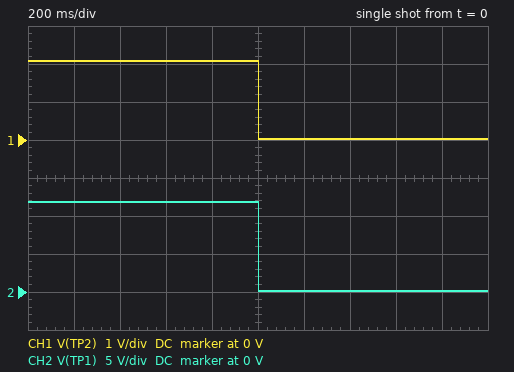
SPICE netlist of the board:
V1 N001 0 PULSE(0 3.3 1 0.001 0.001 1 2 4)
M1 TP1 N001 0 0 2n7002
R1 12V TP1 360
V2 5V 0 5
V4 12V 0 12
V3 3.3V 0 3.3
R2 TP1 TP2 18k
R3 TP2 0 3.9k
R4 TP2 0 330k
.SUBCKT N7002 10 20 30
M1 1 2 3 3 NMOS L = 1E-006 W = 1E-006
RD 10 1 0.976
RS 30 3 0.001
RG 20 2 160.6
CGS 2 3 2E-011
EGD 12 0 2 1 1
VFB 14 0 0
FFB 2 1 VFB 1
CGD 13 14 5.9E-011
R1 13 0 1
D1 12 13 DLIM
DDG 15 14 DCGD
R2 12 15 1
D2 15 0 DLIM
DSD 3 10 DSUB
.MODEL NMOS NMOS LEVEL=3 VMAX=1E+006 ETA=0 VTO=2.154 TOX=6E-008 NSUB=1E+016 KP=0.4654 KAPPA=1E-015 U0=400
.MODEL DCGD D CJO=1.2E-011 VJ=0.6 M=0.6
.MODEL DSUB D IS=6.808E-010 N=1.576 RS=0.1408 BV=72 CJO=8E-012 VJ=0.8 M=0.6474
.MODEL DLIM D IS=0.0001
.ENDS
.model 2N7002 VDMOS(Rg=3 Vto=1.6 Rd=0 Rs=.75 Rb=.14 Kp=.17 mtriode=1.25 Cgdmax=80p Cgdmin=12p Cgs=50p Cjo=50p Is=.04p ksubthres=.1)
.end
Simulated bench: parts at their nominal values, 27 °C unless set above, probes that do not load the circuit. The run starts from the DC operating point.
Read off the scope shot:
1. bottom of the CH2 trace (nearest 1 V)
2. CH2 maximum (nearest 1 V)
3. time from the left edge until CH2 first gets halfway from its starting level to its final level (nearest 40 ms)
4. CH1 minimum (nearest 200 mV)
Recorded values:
0 V
12 V
1.00 s
0 V
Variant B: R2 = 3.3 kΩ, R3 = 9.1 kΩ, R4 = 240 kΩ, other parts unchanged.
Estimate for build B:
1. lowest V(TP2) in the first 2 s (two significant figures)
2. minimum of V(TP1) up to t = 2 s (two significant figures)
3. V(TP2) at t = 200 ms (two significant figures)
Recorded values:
88 mV
120 mV
8.5 V
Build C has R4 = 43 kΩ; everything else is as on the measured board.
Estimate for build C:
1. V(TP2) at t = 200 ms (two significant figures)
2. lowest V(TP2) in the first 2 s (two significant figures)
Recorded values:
2.0 V
20 mV
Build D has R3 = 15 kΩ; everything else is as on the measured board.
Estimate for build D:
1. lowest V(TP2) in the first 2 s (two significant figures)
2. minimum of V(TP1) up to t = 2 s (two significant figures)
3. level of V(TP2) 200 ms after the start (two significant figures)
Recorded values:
54 mV
120 mV
5.3 V
